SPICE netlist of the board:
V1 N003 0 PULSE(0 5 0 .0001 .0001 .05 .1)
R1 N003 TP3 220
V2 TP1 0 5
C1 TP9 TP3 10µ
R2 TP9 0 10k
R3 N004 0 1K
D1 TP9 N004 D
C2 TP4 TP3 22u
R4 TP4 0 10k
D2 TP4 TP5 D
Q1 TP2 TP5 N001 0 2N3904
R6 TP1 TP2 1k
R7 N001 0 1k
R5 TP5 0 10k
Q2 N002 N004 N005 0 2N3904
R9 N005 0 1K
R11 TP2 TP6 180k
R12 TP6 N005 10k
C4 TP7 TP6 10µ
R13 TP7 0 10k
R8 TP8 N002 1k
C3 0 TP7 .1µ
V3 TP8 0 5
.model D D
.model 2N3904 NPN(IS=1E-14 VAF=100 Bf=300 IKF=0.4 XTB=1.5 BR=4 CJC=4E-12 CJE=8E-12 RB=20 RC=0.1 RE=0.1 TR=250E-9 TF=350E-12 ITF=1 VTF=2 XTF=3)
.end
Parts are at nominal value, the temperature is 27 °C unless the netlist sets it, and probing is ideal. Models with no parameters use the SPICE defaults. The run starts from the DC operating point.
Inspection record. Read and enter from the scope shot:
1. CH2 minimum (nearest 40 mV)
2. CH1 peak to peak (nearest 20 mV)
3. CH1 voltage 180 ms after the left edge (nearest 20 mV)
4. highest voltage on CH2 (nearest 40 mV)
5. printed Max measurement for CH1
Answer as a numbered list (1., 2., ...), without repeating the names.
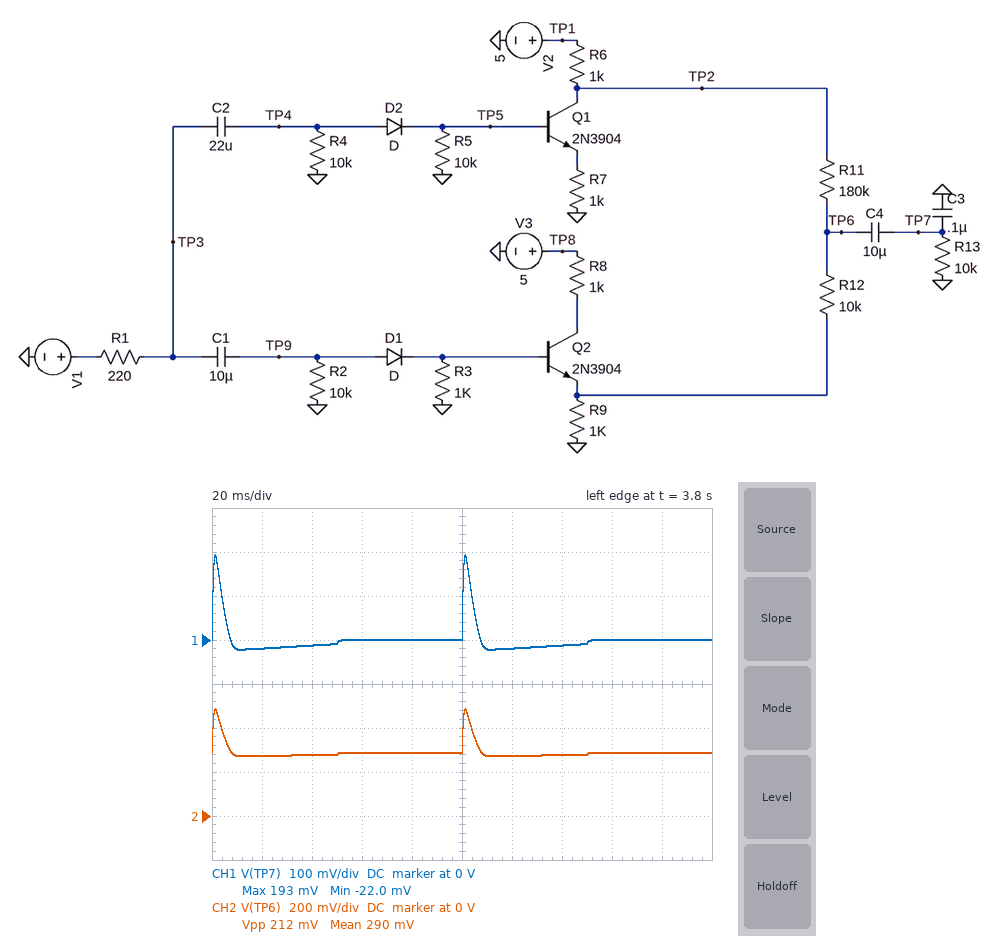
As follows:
1. 280 mV
2. 220 mV
3. 0 V
4. 480 mV
5. 193 mV
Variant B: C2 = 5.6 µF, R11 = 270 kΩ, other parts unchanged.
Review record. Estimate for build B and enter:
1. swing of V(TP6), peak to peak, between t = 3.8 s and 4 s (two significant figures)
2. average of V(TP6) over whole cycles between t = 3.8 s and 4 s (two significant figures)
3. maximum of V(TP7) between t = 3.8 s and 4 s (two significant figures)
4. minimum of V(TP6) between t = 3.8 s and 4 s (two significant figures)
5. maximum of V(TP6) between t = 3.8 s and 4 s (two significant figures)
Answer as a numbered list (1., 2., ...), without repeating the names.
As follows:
1. 190 mV
2. 200 mV
3. 170 mV
4. 180 mV
5. 380 mV
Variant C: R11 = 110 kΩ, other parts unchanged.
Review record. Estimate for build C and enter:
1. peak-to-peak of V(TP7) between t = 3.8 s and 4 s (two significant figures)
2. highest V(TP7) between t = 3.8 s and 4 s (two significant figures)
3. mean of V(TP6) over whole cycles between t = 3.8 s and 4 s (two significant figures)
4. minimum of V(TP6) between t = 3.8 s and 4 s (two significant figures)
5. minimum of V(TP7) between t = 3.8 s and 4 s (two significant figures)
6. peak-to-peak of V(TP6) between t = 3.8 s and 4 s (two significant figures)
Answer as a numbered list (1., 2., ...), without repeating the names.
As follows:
1. 210 mV
2. 180 mV
3. 440 mV
4. 420 mV
5. -28 mV
6. 200 mV
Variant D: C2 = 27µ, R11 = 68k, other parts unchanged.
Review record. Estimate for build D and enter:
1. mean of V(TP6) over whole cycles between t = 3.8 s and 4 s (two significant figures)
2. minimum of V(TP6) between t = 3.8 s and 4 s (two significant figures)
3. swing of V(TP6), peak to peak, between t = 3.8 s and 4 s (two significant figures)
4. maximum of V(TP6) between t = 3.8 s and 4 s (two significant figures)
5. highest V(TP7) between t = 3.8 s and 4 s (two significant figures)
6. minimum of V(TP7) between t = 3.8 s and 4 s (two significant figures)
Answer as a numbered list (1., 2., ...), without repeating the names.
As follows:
1. 670 mV
2. 640 mV
3. 200 mV
4. 830 mV
5. 160 mV
6. -36 mV
